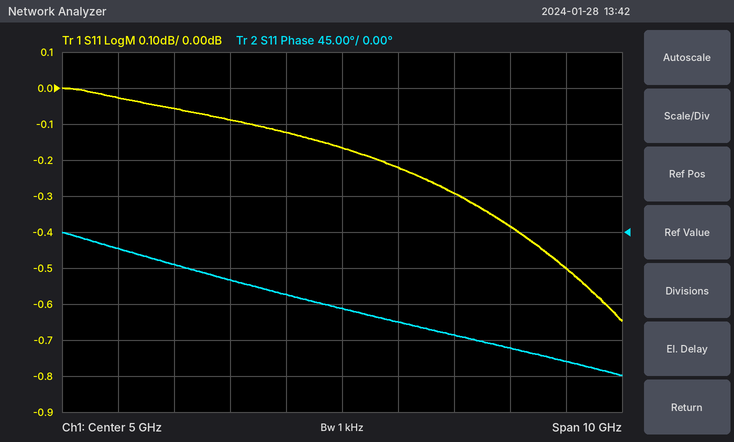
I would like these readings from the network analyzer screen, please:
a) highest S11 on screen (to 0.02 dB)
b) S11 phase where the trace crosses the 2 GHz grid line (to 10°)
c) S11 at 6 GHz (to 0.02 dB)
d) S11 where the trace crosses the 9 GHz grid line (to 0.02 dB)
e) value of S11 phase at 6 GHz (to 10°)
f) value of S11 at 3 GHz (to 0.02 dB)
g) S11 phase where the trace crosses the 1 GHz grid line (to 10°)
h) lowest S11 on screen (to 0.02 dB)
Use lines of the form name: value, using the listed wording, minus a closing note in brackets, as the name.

highest S11 on screen: 0.00 dB
S11 phase where the trace crosses the 2 GHz grid line: -40°
S11 at 6 GHz: -0.22 dB
S11 where the trace crosses the 9 GHz grid line: -0.50 dB
value of S11 phase at 6 GHz: -110°
value of S11 at 3 GHz: -0.08 dB
S11 phase where the trace crosses the 1 GHz grid line: -20°
lowest S11 on screen: -0.64 dB
